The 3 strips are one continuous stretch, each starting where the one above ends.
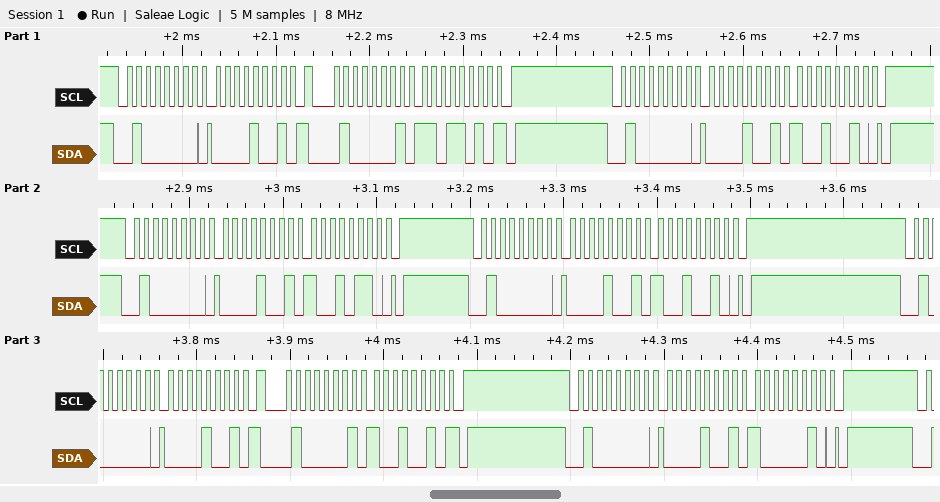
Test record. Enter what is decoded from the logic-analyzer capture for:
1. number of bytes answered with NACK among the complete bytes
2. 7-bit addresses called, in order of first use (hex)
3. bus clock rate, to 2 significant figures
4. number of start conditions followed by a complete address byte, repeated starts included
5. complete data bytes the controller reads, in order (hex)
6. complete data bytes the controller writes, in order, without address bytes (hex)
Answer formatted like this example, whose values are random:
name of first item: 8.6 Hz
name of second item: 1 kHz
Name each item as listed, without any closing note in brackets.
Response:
number of bytes answered with NACK among the complete bytes: 2
7-bit addresses called, in order of first use: 0x20
bus clock rate, to 2 significant figures: 100 kHz
number of start conditions followed by a complete address byte, repeated starts included: 8
complete data bytes the controller reads, in order: DA 92
complete data bytes the controller writes, in order, without address bytes: 09 09 92 09 96 09 92 09 09 82
